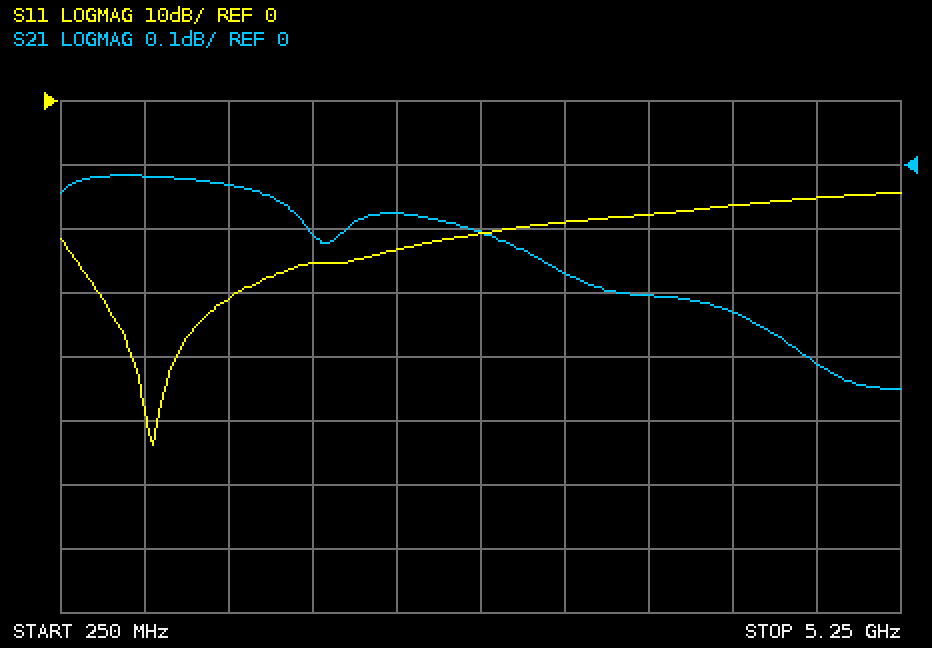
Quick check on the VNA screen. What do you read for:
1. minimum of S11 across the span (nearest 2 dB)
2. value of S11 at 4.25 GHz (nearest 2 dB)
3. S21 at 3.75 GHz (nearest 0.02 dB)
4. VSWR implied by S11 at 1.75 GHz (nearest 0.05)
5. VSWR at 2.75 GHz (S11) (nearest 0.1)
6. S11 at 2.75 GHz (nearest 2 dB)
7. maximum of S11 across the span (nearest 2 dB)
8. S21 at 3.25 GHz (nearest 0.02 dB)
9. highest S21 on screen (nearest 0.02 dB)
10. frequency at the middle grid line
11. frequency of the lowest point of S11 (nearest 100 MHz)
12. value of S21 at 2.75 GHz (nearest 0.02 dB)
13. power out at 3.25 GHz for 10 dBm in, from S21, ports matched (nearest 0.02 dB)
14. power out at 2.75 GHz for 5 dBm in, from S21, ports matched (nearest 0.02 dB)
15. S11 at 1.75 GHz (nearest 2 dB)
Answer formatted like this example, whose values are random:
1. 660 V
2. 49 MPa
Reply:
1. -54 dB
2. -16 dB
3. -0.20 dB
4. 1.10
5. 1.2
6. -20 dB
7. -14 dB
8. -0.16 dB
9. -0.02 dB
10. 2.75 GHz
11. 800 MHz
12. -0.10 dB
13. 9.84 dBm
14. 4.90 dBm
15. -26 dB
